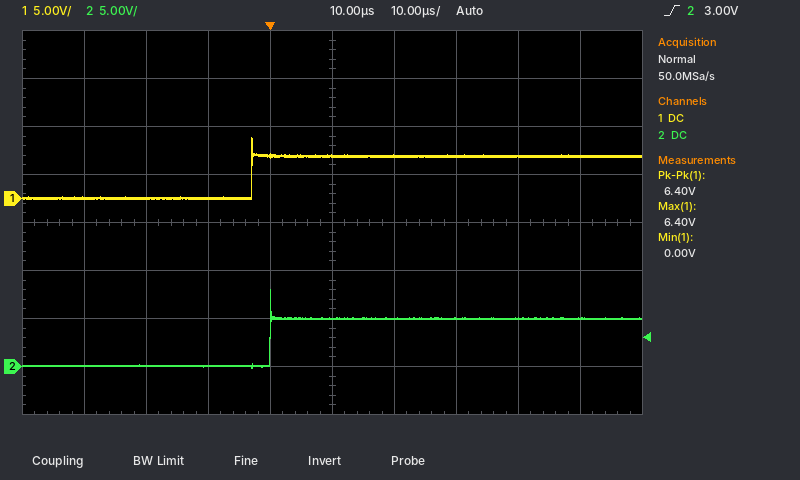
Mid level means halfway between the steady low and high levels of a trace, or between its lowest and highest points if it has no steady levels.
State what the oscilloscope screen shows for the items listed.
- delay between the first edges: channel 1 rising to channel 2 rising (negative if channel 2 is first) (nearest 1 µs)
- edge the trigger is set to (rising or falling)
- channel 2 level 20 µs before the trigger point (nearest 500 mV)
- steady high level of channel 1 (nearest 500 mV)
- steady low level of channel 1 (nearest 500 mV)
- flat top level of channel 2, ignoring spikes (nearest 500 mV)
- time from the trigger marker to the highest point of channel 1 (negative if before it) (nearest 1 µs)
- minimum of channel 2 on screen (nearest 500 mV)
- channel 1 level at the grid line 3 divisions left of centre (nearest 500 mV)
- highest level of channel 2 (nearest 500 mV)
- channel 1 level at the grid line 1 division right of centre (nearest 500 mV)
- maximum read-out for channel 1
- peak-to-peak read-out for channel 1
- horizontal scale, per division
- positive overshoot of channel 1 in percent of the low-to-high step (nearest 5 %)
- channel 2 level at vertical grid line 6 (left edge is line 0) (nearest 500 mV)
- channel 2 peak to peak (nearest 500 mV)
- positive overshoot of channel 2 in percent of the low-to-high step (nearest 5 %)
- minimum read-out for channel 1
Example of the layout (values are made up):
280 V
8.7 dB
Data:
+3 µs
rising
0.0 V
4.5 V
0.0 V
5.0 V
-3 µs
0.0 V
0.0 V
8.0 V
4.5 V
6.40 V
6.40 V
10 µs
45 %
5.0 V
8.0 V
60 %
0.00 V
